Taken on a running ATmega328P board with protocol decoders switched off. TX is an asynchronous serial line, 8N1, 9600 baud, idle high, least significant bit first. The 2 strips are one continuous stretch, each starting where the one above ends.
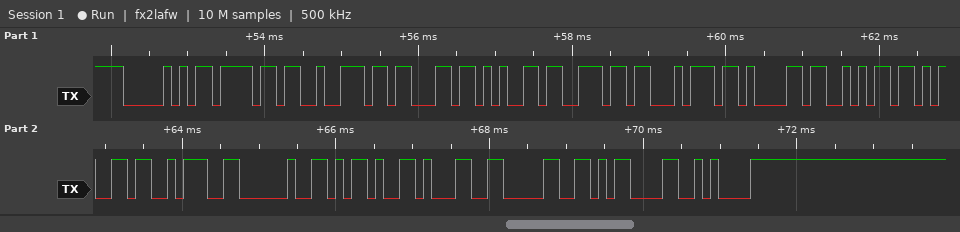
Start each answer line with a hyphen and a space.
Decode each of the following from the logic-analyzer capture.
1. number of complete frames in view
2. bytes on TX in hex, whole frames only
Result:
- 17
- 50 6F 72 63 65 6E 74 61 6A 65 3A 20 2D 31 30 0D 0A
